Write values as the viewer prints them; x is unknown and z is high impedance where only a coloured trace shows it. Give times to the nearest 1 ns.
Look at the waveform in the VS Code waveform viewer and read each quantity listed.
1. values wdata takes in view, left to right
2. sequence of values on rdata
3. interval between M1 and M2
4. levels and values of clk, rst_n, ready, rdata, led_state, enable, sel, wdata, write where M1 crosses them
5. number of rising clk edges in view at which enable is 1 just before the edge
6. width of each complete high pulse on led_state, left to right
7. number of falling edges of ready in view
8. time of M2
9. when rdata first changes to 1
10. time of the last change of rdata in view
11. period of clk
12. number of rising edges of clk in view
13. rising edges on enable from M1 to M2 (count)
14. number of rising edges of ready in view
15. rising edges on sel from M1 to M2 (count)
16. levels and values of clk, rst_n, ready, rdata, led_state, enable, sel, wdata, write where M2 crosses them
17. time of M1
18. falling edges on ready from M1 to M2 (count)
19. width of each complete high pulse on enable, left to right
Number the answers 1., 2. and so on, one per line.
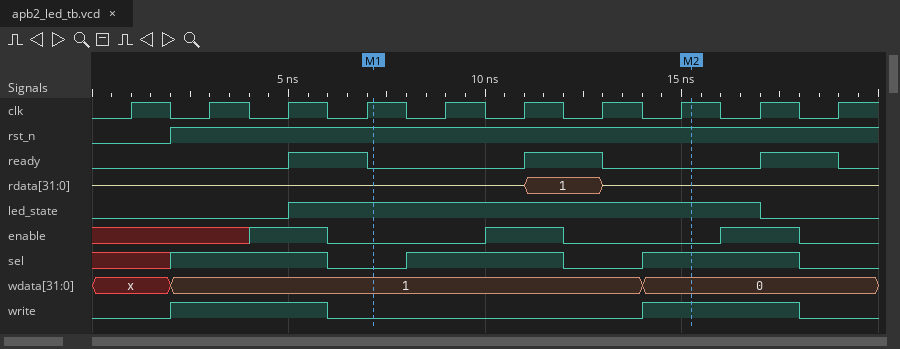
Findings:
1. x, 1, 0
2. z, 1, z
3. 8 ns
4. clk=1, rst_n=1, ready=0, rdata=z, led_state=1, enable=0, sel=0, wdata=1, write=0
5. 3
6. 12 ns
7. 3
8. 15 ns
9. 11 ns
10. 13 ns
11. 2 ns
12. 10
13. 1
14. 3
15. 2
16. clk=1, rst_n=1, ready=0, rdata=z, led_state=1, enable=0, sel=1, wdata=0, write=1
17. 7 ns
18. 1
19. 2 ns, 2 ns
